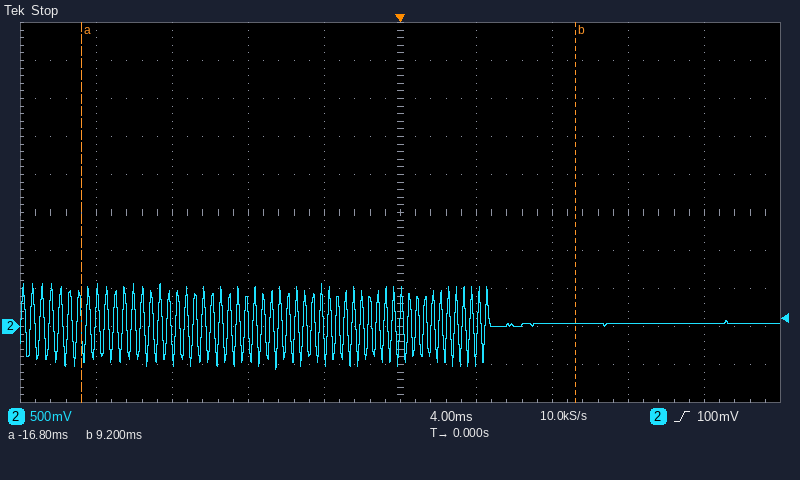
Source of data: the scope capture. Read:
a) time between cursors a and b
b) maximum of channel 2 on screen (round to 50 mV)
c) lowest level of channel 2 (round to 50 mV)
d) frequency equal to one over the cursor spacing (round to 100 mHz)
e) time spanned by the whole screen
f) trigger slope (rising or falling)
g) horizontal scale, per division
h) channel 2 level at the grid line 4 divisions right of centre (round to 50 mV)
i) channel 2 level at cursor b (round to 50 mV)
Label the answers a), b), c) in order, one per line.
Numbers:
a) 26.0 ms
b) 550 mV
c) -550 mV
d) 38.5 Hz
e) 40 ms
f) rising
g) 4 ms
h) 50 mV
i) 50 mV
